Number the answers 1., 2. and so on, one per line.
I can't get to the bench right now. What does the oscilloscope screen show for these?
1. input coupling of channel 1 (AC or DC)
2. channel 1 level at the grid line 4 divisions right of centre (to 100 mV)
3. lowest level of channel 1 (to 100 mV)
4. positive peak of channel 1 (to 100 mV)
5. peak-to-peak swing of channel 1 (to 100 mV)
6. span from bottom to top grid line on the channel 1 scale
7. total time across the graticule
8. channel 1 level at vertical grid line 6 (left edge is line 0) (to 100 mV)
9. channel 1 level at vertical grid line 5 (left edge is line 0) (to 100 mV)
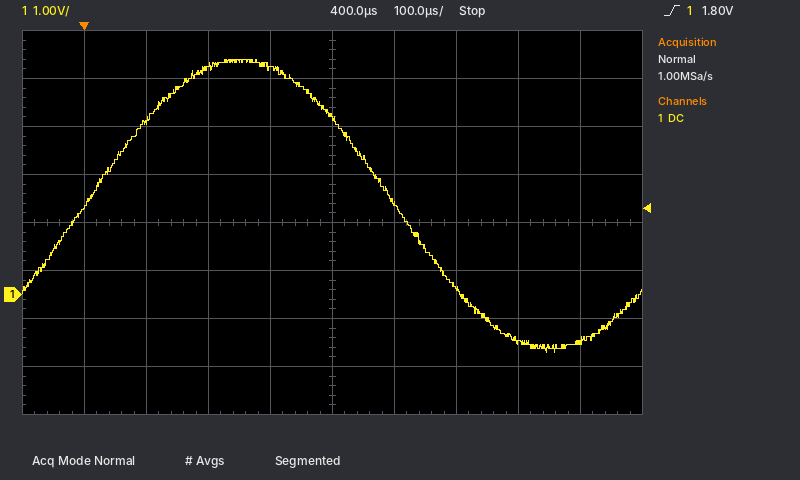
1. DC
2. -1.0 V
3. -1.2 V
4. 4.9 V
5. 6.1 V
6. 8 V
7. 1 ms
8. 1.9 V
9. 3.7 V
